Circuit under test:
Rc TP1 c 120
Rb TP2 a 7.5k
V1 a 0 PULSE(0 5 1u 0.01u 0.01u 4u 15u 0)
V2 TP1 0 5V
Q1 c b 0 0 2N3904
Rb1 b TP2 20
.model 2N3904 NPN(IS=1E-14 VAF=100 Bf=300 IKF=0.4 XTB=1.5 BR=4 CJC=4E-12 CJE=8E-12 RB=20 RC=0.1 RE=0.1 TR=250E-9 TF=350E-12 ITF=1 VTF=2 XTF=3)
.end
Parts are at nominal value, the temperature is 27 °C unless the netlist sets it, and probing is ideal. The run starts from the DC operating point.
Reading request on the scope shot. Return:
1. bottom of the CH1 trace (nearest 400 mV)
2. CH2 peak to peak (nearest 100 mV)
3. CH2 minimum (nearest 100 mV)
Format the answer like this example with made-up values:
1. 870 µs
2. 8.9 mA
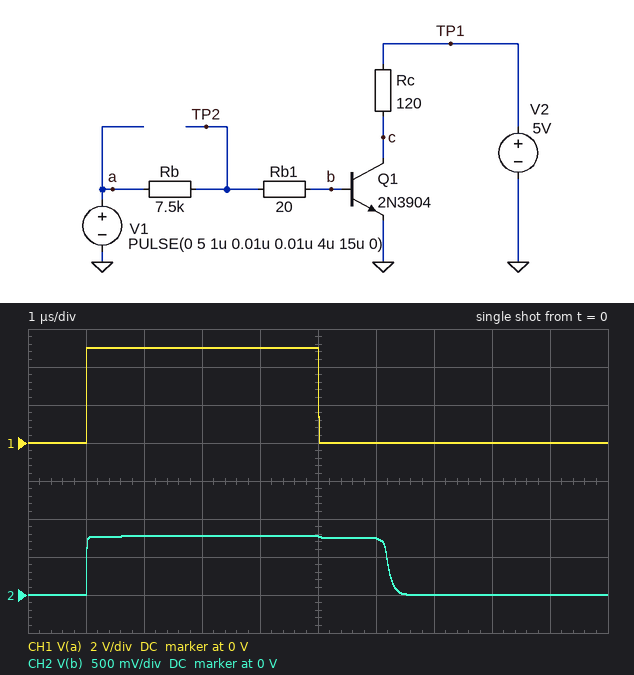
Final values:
1. 0 V
2. 800 mV
3. 0 V
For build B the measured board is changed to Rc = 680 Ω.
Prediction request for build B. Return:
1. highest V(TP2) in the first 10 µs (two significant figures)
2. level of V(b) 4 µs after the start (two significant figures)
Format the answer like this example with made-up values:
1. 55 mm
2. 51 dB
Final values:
1. 740 mV
2. 730 mV
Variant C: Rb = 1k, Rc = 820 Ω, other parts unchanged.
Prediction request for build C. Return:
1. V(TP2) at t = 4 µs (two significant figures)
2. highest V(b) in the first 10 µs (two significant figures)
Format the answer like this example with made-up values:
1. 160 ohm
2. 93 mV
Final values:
1. 900 mV
2. 820 mV
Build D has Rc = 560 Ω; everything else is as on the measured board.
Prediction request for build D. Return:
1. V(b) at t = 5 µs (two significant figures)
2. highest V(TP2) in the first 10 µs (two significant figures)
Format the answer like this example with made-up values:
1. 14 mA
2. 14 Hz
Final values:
1. 730 mV
2. 740 mV
